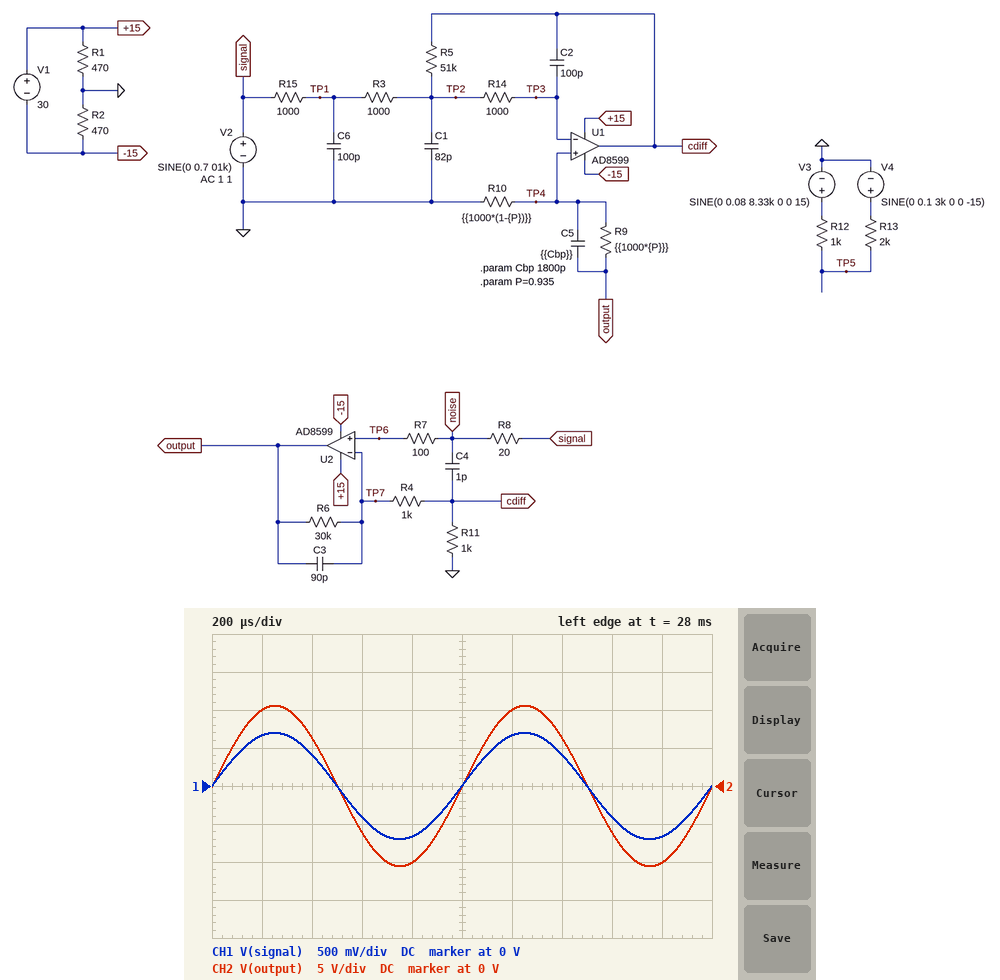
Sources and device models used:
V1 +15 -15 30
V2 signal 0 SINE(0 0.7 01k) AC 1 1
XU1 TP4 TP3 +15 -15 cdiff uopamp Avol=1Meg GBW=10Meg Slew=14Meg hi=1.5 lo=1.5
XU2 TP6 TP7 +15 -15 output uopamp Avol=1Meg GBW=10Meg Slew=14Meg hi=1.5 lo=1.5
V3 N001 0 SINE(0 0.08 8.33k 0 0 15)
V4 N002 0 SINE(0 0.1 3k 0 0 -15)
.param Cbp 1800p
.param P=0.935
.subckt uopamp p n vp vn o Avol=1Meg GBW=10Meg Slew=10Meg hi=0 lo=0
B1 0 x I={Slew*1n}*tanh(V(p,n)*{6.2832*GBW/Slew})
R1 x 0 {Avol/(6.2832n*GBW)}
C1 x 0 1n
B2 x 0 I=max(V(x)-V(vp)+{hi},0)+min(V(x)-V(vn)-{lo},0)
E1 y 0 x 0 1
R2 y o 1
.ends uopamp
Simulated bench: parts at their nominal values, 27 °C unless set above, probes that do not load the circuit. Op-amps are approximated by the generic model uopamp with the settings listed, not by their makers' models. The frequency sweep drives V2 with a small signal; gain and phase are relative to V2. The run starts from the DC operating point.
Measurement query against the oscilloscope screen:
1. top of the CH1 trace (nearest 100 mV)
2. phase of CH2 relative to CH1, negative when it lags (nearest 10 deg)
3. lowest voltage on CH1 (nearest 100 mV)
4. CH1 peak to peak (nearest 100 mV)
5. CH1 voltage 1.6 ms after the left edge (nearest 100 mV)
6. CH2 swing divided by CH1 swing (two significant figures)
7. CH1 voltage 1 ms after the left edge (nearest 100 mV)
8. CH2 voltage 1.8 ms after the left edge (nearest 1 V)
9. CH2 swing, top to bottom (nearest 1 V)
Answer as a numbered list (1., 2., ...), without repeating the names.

1. 700 mV
2. 0 deg
3. -700 mV
4. 1.4 V
5. -400 mV
6. 15
7. 0 V
8. -10 V
9. 21 V
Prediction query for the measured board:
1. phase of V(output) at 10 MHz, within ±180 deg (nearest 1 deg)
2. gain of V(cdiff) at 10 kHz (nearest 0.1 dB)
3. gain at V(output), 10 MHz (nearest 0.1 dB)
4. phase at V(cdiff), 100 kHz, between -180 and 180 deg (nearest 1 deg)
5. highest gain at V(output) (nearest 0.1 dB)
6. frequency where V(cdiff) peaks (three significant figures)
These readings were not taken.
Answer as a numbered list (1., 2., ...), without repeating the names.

1. -50 deg
2. -5.6 dB
3. -3.0 dB
4. -2 deg
5. 23.6 dB
6. 2.62 MHz
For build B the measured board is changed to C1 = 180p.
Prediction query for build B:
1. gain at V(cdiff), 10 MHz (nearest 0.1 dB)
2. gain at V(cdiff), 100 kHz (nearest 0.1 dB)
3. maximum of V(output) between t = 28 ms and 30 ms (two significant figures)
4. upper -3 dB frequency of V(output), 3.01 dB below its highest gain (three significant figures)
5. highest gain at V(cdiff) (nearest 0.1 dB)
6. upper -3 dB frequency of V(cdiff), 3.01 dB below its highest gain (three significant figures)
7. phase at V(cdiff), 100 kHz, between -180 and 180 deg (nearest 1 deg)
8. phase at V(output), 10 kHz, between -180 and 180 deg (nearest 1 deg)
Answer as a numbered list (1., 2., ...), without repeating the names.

1. -6.6 dB
2. -9.4 dB
3. 11 V
4. 82.7 kHz
5. 0.8 dB
6. 5.53 MHz
7. 10 deg
8. -8 deg
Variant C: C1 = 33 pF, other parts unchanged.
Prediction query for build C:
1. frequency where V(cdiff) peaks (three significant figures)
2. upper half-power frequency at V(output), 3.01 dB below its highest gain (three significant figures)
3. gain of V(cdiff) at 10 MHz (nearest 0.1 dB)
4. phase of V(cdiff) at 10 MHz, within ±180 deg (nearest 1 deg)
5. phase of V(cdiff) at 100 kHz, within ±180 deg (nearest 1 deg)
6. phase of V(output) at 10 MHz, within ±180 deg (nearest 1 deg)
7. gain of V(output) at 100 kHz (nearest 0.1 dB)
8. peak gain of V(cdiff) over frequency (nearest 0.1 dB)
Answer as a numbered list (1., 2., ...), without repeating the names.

1. 2.97 MHz
2. 90.9 kHz
3. -6.3 dB
4. -92 deg
5. -10 deg
6. -50 deg
7. 20.1 dB
8. 0 dB
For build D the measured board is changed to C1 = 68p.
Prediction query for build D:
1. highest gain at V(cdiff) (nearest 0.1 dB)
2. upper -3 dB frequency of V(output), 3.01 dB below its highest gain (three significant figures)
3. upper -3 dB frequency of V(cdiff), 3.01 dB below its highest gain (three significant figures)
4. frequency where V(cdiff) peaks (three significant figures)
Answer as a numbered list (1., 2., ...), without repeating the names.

1. 0.4 dB
2. 89.0 kHz
3. 6.23 MHz
4. 2.71 MHz
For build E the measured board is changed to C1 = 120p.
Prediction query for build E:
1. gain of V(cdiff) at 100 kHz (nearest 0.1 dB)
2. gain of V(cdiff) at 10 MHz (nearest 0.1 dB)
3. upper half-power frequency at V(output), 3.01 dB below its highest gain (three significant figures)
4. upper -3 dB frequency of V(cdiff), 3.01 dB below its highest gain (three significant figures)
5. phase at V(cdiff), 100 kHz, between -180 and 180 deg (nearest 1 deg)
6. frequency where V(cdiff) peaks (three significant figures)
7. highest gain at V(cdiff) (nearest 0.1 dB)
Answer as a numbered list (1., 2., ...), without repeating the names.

1. -10.1 dB
2. -6.6 dB
3. 86.0 kHz
4. 5.78 MHz
5. 3 deg
6. 2.41 MHz
7. 0.7 dB
